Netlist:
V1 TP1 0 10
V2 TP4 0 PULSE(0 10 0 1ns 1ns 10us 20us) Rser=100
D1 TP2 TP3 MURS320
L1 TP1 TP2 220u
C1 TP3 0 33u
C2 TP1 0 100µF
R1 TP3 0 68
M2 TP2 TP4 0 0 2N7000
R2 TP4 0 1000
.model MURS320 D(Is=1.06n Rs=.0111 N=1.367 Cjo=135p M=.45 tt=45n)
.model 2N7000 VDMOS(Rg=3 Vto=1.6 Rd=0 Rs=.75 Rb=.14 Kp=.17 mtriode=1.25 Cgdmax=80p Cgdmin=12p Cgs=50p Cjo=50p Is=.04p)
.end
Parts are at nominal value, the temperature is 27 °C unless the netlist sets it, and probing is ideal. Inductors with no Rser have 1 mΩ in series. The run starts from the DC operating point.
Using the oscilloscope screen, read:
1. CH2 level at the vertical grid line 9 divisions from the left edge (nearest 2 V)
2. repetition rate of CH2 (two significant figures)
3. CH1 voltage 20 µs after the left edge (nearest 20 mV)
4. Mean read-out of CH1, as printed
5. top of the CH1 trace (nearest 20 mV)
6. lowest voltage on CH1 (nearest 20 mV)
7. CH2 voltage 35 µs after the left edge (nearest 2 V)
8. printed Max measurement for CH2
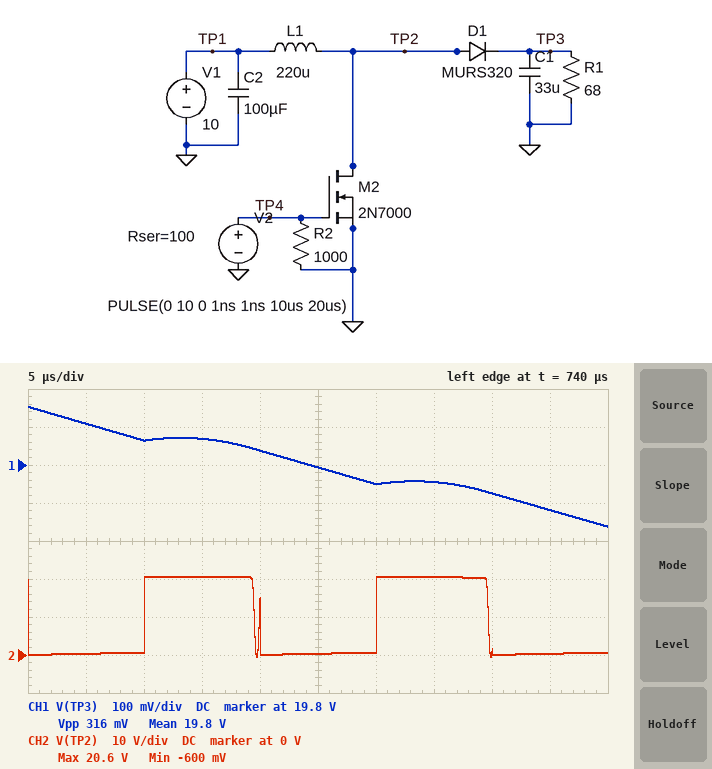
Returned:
0 V
100 kHz
19.84 V
19.8 V
19.96 V
19.64 V
20 V
20.6 V
